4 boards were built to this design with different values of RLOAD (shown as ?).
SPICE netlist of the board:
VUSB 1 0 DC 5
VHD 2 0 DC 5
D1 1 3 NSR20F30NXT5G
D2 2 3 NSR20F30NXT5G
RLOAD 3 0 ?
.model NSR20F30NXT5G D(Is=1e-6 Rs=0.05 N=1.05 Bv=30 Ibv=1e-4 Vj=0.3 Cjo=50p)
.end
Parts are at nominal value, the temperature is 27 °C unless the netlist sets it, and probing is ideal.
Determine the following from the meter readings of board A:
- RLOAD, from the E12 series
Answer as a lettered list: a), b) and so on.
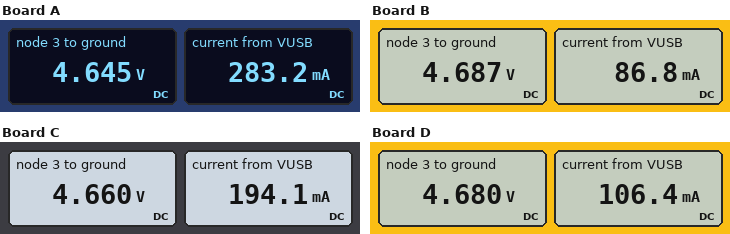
a) 8.2 Ω
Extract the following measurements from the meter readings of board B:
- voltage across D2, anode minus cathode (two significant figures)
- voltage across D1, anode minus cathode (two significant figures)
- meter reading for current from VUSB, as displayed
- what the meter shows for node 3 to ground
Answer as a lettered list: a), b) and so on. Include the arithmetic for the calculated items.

a) 5 V - 4.687 V = 310 mV
b) 5 V - 4.687 V = 310 mV
c) 86.8 mA
d) 4.687 V
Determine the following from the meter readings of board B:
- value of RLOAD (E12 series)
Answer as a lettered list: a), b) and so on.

a) 27 Ω
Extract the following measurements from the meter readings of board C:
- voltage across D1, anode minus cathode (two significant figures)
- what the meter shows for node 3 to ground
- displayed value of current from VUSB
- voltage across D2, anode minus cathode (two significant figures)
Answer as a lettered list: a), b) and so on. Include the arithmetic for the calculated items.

a) 5 V - 4.66 V = 340 mV
b) 4.660 V
c) 194.1 mA
d) 5 V - 4.66 V = 340 mV
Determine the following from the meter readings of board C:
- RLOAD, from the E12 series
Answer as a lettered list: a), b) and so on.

a) 12 Ω
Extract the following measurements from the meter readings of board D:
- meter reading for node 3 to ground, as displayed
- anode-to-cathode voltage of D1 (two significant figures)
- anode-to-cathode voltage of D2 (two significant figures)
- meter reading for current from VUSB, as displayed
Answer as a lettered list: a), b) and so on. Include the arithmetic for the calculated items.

a) 4.680 V
b) 5 V - 4.68 V = 320 mV
c) 5 V - 4.68 V = 320 mV
d) 106.4 mA
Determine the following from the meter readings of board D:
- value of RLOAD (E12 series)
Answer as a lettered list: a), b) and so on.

a) 22 Ω
